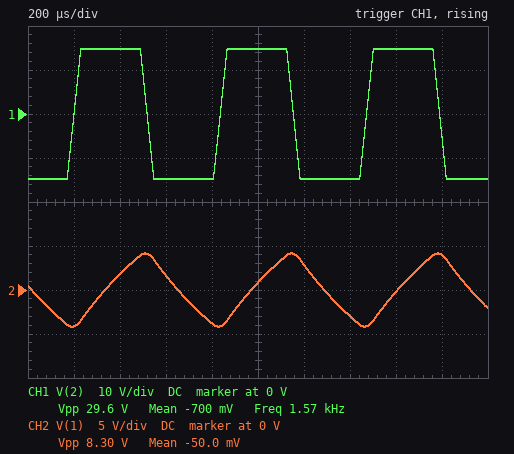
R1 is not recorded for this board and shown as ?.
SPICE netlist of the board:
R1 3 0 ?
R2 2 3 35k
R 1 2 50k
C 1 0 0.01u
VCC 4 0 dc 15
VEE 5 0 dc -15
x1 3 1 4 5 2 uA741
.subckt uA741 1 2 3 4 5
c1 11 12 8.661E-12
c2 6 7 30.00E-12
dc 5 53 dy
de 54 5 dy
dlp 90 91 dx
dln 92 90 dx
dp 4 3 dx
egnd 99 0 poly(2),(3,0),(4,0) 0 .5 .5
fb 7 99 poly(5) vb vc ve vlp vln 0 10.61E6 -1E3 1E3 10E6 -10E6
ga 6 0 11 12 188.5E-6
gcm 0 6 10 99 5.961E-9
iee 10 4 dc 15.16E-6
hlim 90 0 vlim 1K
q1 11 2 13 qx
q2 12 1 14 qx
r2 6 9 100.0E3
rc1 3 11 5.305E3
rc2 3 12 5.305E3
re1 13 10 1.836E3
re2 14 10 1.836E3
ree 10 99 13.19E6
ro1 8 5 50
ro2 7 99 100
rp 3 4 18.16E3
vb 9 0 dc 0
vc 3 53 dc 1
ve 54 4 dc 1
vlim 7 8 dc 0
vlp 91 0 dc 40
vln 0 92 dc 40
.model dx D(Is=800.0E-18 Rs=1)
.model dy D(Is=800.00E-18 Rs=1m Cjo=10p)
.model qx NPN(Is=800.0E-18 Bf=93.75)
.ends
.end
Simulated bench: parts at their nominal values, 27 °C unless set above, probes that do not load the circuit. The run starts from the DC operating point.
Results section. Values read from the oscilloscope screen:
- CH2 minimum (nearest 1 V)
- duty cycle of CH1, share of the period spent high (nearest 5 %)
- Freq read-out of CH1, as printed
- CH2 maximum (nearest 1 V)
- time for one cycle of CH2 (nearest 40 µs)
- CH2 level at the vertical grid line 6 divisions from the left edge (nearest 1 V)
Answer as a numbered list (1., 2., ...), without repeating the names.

1. -4 V
2. 50 %
3. 1.57 kHz
4. 4 V
5. 640 µs
6. 3 V
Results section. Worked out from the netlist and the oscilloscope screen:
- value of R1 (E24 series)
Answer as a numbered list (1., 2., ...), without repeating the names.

1. 12 kΩ
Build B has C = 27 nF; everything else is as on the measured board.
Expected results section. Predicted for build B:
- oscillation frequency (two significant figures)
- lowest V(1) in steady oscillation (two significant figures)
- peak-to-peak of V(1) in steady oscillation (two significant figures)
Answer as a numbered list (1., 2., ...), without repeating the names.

1. 650 Hz
2. -3.9 V
3. 7.9 V
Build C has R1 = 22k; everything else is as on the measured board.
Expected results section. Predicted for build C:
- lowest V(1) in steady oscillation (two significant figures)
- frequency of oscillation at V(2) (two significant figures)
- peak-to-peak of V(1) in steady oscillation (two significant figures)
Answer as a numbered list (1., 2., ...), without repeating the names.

1. -6.0 V
2. 1.1 kHz
3. 12 V
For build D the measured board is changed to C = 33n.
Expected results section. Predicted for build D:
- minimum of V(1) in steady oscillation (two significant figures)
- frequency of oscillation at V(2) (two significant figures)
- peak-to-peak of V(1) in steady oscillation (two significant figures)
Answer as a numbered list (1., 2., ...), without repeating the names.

1. -3.9 V
2. 540 Hz
3. 7.8 V
